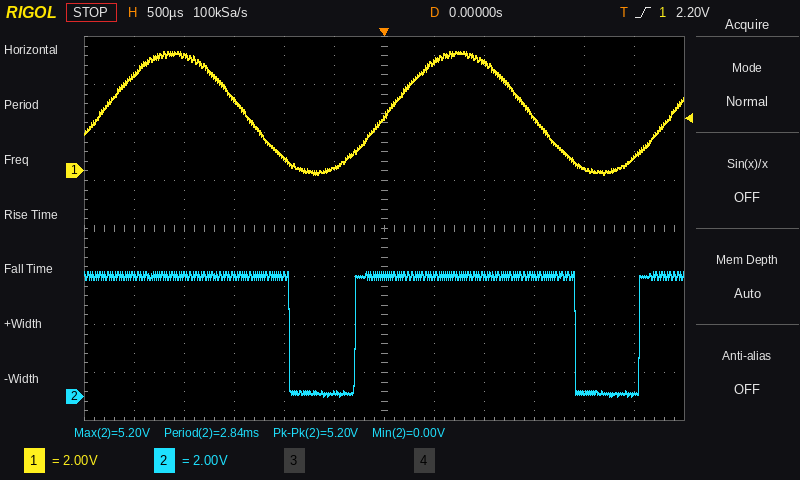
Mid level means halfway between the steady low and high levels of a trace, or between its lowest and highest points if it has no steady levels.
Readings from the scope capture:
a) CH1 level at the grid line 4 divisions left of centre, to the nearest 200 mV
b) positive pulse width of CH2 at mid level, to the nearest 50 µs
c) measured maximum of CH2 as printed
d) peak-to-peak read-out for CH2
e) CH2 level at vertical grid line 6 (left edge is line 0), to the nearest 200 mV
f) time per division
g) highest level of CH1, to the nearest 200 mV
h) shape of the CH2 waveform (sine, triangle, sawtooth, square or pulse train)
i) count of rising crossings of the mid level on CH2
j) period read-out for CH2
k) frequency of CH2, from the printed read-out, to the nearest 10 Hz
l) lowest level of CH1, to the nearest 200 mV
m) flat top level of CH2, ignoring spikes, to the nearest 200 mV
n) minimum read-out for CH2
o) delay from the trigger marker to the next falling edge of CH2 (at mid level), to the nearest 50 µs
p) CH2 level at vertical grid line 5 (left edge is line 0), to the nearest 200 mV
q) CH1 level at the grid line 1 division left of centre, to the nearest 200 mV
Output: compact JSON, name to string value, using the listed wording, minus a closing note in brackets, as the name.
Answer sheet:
{"CH1 level at the grid line 4 divisions left of centre, to the nearest 200 mV": "4.8 V", "positive pulse width of CH2 at mid level, to the nearest 50 µs": "2.20 ms", "measured maximum of CH2 as printed": "5.20 V", "peak-to-peak read-out for CH2": "5.20 V", "CH2 level at vertical grid line 6 (left edge is line 0), to the nearest 200 mV": "5.0 V", "time per division": "500 µs", "highest level of CH1, to the nearest 200 mV": "5.0 V", "shape of the CH2 waveform": "pulse train", "count of rising crossings of the mid level on CH2": "2", "period read-out for CH2": "2.84 ms", "frequency of CH2, from the printed read-out, to the nearest 10 Hz": "350 Hz", "lowest level of CH1, to the nearest 200 mV": "-200 mV", "flat top level of CH2, ignoring spikes, to the nearest 200 mV": "5.0 V", "minimum read-out for CH2": "0.00 V", "delay from the trigger marker to the next falling edge of CH2 (at mid level), to the nearest 50 µs": "1.90 ms", "CH2 level at vertical grid line 5 (left edge is line 0), to the nearest 200 mV": "200 mV", "CH1 level at the grid line 1 division left of centre, to the nearest 200 mV": "200 mV"}
